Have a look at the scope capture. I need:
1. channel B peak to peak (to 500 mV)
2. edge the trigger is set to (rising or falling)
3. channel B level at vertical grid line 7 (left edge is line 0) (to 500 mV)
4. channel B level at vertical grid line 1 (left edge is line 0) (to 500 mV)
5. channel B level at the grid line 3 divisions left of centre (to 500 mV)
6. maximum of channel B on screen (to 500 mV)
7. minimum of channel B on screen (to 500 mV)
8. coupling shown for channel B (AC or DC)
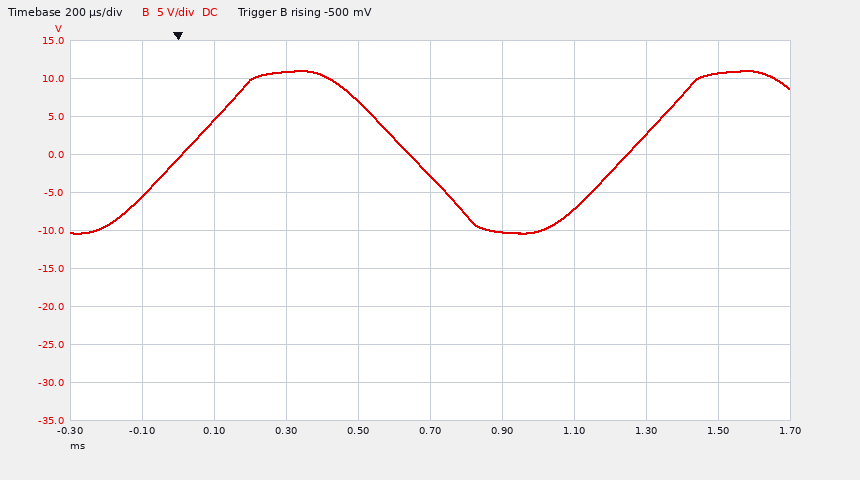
21.5 V
rising
-7.0 V
-5.5 V
4.5 V
11.0 V
-10.5 V
DC
